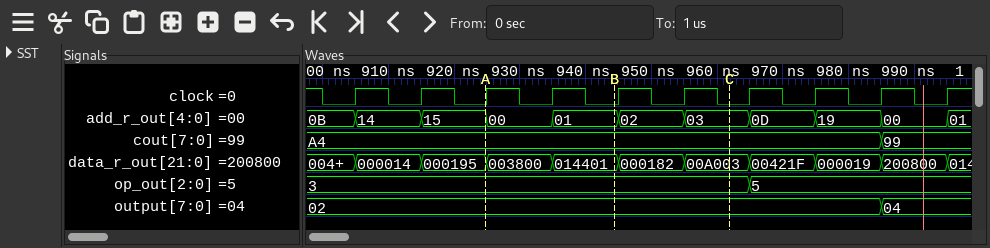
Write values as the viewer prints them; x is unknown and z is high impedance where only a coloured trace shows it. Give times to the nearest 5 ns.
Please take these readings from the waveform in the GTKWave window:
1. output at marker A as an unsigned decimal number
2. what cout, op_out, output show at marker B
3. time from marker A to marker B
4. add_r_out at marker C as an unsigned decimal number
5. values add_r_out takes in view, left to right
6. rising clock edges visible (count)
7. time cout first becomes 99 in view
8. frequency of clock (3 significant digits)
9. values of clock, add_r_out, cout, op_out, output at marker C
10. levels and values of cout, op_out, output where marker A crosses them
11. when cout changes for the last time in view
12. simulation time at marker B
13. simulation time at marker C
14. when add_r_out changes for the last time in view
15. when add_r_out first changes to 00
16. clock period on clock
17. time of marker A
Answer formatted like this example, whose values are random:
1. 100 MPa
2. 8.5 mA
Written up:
1. 2
2. cout=A4, op_out=3, output=02
3. 20 ns
4. 3
5. 0B, 14, 15, 00, 01, 02, 03, 0D, 19, 00, 01
6. 10
7. 985 ns
8. 100 MHz
9. clock=0, add_r_out=03, cout=A4, op_out=3, output=02
10. cout=A4, op_out=3, output=02
11. 985 ns
12. 945 ns
13. 960 ns
14. 995 ns
15. 925 ns
16. 10 ns
17. 925 ns
